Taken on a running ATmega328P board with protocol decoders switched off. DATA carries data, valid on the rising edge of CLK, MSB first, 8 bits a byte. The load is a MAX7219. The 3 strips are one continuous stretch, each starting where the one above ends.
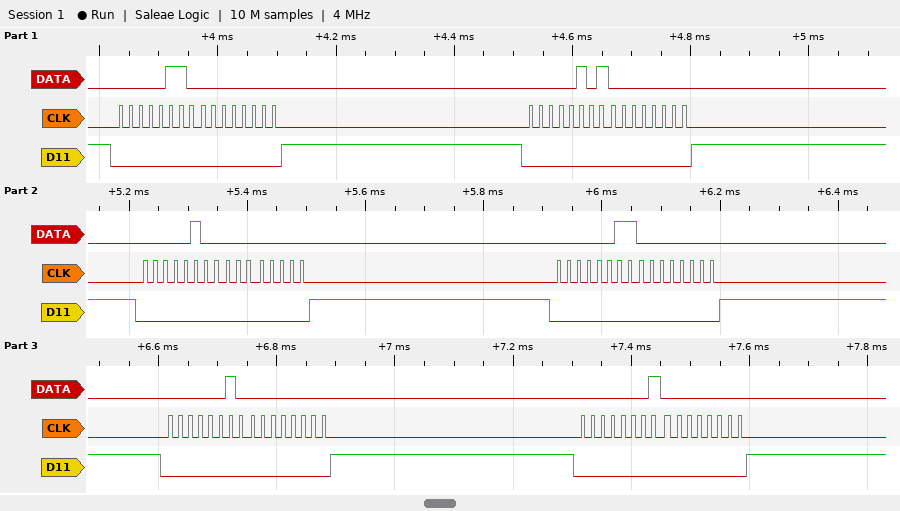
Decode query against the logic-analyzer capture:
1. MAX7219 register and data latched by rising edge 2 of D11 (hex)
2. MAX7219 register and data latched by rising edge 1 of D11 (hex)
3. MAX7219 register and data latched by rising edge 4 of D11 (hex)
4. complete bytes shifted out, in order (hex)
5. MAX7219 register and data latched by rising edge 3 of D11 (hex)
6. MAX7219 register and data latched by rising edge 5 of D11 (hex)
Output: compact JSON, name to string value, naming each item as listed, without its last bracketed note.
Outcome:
{"MAX7219 register and data latched by rising edge 2 of D11": "register 0x5, data 0x00", "MAX7219 register and data latched by rising edge 1 of D11": "register 0x6, data 0x00", "MAX7219 register and data latched by rising edge 4 of D11": "register 0x3, data 0x00", "complete bytes shifted out, in order": "06 00 05 00 04 00 03 00 02 00 01 00", "MAX7219 register and data latched by rising edge 3 of D11": "register 0x4, data 0x00", "MAX7219 register and data latched by rising edge 5 of D11": "register 0x2, data 0x00"}
